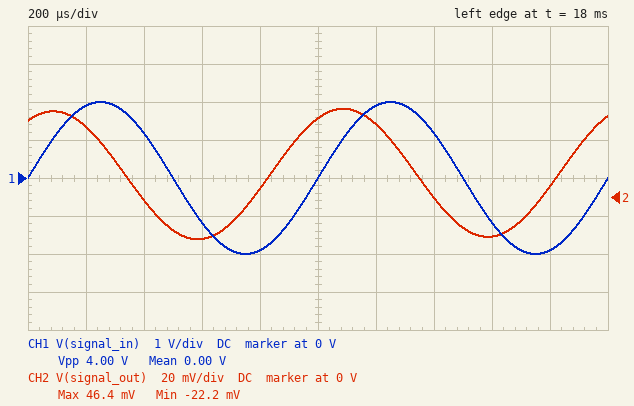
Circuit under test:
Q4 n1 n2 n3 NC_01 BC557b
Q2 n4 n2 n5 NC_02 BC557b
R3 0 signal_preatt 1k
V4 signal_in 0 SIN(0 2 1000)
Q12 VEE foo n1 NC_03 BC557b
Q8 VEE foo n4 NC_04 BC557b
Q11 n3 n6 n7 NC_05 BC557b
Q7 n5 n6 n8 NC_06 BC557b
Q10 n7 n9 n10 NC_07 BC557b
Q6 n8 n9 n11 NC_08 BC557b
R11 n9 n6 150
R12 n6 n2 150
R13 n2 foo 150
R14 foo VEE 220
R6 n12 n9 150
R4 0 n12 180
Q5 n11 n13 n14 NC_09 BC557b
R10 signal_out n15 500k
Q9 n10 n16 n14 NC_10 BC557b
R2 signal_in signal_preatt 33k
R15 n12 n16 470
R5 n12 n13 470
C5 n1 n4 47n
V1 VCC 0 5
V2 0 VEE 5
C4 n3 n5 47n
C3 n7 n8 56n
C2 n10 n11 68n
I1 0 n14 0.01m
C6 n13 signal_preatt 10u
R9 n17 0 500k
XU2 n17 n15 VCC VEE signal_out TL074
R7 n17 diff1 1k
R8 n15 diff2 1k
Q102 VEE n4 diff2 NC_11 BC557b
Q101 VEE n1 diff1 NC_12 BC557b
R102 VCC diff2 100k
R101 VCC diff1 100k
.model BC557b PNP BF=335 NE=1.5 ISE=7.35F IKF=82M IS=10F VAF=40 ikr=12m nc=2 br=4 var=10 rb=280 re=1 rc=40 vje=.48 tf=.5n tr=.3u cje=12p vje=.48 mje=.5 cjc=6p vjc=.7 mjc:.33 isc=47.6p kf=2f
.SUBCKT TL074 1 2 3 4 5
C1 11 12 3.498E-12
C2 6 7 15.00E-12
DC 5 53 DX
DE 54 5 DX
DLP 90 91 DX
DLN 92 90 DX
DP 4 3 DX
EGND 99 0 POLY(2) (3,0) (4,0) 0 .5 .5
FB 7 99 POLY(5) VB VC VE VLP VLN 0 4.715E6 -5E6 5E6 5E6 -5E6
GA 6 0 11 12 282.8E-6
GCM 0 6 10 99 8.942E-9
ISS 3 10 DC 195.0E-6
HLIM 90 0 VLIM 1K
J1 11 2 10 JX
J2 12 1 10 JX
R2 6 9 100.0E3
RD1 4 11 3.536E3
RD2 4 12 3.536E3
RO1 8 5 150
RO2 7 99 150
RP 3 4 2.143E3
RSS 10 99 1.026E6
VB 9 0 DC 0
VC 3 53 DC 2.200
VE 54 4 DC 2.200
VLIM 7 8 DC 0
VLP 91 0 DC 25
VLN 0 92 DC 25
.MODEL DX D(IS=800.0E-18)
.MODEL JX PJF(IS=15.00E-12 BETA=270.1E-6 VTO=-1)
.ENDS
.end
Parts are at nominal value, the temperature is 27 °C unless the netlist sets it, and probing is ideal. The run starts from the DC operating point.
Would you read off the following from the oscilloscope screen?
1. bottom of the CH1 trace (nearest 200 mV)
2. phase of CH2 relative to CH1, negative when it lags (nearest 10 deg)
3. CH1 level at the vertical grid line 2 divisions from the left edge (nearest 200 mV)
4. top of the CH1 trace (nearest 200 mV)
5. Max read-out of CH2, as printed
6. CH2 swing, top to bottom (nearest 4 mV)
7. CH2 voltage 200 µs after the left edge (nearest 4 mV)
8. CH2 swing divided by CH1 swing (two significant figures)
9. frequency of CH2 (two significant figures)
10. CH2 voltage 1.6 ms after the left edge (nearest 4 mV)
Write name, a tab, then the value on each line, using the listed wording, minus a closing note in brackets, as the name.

bottom of the CH1 trace	-2.0 V
phase of CH2 relative to CH1, negative when it lags	60 deg
CH1 level at the vertical grid line 2 divisions from the left edge	1.2 V
top of the CH1 trace	2.0 V
Max read-out of CH2, as printed	46.4 mV
CH2 swing, top to bottom	68 mV
CH2 voltage 200 µs after the left edge	36 mV
CH2 swing divided by CH1 swing	0.017
frequency of CH2	1.0 kHz
CH2 voltage 1.6 ms after the left edge	-20 mV
